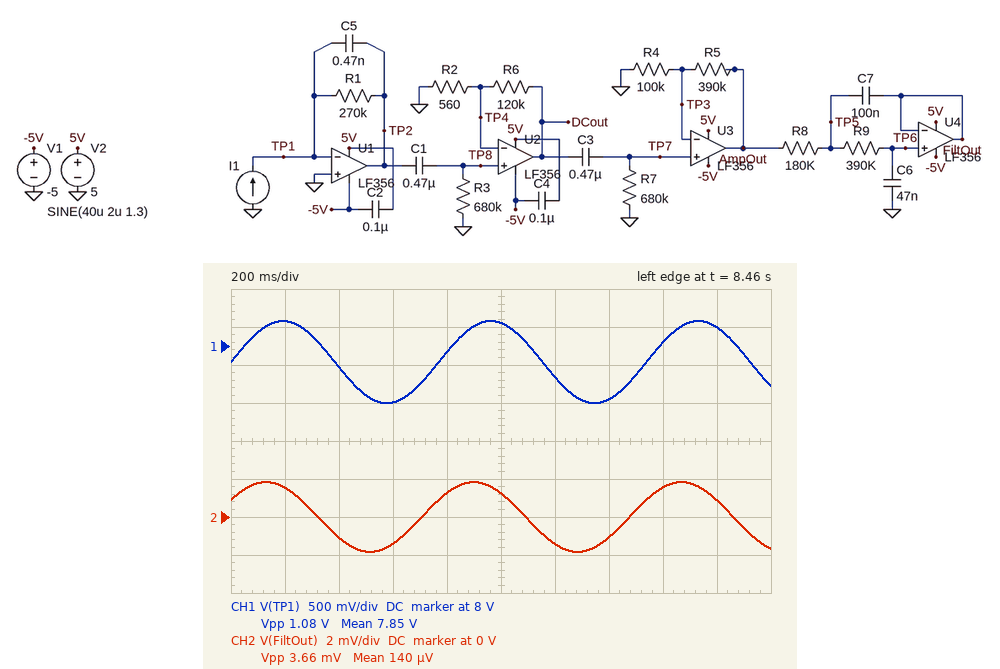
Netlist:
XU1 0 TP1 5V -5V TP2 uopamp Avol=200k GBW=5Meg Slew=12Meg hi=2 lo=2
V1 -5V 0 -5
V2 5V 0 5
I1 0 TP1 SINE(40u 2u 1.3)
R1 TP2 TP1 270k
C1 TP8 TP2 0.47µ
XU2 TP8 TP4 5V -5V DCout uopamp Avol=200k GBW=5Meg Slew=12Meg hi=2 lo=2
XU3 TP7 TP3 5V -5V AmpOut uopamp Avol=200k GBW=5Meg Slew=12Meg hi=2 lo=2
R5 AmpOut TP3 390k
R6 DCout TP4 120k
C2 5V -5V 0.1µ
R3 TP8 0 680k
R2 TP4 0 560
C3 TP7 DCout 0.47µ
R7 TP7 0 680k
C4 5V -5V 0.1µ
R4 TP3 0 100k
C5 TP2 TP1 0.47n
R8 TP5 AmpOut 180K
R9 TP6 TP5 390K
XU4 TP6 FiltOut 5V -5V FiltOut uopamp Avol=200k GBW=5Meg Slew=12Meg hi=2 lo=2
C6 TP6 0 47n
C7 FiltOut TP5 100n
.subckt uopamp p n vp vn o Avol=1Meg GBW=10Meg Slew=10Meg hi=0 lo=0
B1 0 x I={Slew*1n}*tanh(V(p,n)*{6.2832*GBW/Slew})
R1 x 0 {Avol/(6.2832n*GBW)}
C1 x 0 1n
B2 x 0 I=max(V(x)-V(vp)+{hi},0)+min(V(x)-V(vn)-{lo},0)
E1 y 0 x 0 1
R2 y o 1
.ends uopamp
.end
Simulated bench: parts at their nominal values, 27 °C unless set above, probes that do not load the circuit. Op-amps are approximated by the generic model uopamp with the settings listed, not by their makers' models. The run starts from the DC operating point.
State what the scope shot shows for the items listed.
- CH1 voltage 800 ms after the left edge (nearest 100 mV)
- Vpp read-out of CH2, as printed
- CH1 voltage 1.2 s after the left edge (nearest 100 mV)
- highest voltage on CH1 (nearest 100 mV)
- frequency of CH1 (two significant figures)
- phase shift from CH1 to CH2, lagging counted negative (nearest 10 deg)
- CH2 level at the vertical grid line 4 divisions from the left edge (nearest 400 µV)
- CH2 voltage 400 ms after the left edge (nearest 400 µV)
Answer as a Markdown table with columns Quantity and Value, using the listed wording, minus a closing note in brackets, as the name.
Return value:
| Quantity | Value |
|---|---|
| CH1 voltage 800 ms after the left edge | 7.9 V |
| Vpp read-out of CH2, as printed | 3.66 mV |
| CH1 voltage 1.2 s after the left edge | 7.6 V |
| highest voltage on CH1 | 8.3 V |
| frequency of CH1 | 1.3 Hz |
| phase shift from CH1 to CH2, lagging counted negative | 30 deg |
| CH2 level at the vertical grid line 4 divisions from the left edge | 1.2 mV |
| CH2 voltage 400 ms after the left edge | -1.2 mV |
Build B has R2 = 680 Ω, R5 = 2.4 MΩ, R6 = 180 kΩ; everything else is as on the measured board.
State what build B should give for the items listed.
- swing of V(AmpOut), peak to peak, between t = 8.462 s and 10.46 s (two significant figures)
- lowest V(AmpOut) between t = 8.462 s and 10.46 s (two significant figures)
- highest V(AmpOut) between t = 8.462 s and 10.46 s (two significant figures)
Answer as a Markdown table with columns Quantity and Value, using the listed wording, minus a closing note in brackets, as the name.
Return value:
| Quantity | Value |
|---|---|
| swing of V(AmpOut), peak to peak, between t = 8.462 s and 10.46 s | 23 mV |
| lowest V(AmpOut) between t = 8.462 s and 10.46 s | -12 mV |
| highest V(AmpOut) between t = 8.462 s and 10.46 s | 12 mV |
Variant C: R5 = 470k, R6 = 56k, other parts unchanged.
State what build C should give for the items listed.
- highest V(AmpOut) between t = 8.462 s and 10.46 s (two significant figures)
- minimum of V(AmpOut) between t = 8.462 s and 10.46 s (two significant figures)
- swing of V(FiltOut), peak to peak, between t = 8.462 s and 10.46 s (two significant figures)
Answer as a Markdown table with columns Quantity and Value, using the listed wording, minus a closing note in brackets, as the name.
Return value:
| Quantity | Value |
|---|---|
| highest V(AmpOut) between t = 8.462 s and 10.46 s | 1.0 mV |
| minimum of V(AmpOut) between t = 8.462 s and 10.46 s | -1.0 mV |
| swing of V(FiltOut), peak to peak, between t = 8.462 s and 10.46 s | 2.0 mV |
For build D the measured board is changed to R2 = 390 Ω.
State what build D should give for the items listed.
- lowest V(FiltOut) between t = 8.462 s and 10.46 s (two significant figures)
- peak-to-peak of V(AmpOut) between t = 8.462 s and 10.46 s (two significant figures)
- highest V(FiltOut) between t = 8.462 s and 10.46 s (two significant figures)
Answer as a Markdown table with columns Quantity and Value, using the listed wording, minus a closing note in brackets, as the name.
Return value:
| Quantity | Value |
|---|---|
| lowest V(FiltOut) between t = 8.462 s and 10.46 s | -2.6 mV |
| peak-to-peak of V(AmpOut) between t = 8.462 s and 10.46 s | 5.3 mV |
| highest V(FiltOut) between t = 8.462 s and 10.46 s | 2.6 mV |
